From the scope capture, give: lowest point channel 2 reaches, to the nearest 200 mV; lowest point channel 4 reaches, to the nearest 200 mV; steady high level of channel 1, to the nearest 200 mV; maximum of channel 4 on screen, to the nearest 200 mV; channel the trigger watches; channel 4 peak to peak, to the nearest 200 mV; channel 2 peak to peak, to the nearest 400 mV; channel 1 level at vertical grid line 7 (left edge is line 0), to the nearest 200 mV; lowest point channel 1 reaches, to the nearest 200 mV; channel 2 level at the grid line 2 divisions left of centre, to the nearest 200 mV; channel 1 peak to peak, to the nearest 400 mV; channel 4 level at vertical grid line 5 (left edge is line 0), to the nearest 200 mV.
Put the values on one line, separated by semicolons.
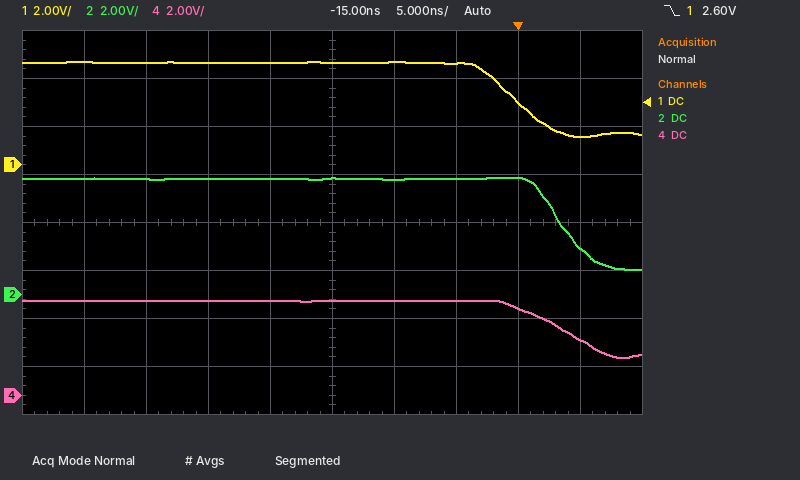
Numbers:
1.0 V; 1.6 V; 4.2 V; 4.0 V; channel 1; 2.4 V; 4.0 V; 4.2 V; 1.2 V; 4.8 V; 3.2 V; 4.0 V
